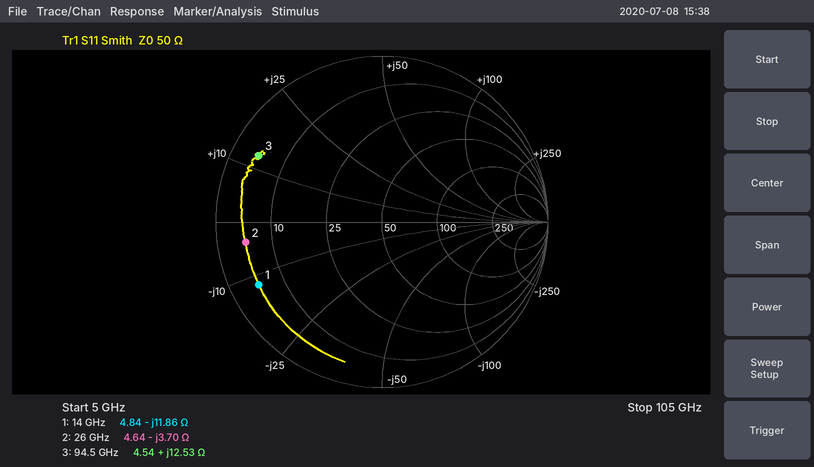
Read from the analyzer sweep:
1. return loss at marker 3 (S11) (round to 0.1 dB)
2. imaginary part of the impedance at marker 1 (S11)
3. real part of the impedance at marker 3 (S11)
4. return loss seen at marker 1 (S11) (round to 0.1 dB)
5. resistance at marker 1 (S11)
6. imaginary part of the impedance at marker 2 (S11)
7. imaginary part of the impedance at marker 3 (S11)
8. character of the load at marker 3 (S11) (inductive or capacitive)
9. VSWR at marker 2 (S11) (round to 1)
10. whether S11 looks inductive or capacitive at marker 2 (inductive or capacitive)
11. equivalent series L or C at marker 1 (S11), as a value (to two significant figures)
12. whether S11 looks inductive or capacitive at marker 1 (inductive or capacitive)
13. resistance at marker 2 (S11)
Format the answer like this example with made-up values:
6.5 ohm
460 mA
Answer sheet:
1.5 dB
-11.86 Ω
4.54 Ω
1.6 dB
4.84 Ω
-3.70 Ω
+12.53 Ω
inductive
11
capacitive
960 fF
capacitive
4.64 Ω
